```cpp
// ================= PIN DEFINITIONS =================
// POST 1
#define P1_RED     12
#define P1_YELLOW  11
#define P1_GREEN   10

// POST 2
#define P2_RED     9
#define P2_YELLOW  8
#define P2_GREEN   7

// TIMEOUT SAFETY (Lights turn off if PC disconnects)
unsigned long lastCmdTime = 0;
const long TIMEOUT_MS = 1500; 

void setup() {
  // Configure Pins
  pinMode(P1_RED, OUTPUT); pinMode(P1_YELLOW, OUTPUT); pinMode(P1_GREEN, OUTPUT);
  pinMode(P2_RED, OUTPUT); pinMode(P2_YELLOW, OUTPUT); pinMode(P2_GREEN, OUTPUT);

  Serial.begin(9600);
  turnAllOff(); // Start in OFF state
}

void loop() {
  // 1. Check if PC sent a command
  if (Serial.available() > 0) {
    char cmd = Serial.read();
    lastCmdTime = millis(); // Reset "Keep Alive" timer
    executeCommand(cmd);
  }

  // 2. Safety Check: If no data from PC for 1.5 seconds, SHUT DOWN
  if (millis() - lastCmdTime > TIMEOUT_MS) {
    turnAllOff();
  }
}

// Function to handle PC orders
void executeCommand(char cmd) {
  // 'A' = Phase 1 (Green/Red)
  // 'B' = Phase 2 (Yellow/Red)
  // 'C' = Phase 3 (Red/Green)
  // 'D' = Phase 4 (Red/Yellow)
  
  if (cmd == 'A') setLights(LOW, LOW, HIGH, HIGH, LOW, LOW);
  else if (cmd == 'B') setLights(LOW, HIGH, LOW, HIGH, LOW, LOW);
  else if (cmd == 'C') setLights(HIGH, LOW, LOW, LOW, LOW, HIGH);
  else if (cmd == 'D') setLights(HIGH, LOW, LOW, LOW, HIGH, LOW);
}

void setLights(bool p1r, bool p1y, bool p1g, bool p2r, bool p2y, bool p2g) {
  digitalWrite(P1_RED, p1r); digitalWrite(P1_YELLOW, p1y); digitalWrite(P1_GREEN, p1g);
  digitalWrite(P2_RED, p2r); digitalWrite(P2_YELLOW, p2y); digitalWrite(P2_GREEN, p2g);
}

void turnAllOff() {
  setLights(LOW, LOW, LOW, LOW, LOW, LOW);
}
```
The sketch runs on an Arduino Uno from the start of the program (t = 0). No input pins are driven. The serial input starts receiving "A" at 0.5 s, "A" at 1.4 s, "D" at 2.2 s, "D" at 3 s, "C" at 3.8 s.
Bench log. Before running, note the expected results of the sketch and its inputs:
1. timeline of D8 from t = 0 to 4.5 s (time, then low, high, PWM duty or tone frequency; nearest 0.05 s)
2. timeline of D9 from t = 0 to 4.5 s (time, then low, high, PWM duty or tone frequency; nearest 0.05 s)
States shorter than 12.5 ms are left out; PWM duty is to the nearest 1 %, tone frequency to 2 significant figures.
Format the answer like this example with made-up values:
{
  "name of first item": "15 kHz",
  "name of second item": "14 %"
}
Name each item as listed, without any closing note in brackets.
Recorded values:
{
  "timeline of D8 from t = 0 to 4.5 s": "0 s low; 2.2 s high; 3.8 s low",
  "timeline of D9 from t = 0 to 4.5 s": "0 s low; 0.5 s high; 2.2 s low"
}
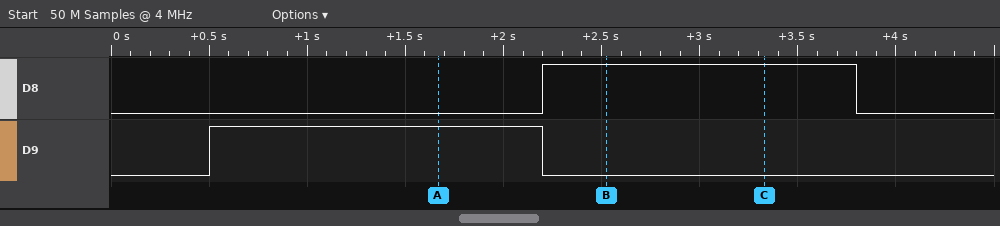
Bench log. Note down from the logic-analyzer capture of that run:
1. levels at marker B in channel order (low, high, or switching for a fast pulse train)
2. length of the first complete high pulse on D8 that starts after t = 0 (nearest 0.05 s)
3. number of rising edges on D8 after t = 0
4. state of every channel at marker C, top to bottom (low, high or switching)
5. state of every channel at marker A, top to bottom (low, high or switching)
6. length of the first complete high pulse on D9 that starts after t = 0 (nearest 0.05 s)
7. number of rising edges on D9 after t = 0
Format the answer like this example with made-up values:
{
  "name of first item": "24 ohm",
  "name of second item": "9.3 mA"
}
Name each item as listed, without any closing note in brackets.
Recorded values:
{
  "levels at marker B in channel order": "D8 high, D9 low",
  "length of the first complete high pulse on D8 that starts after t = 0": "1.60 s",
  "number of rising edges on D8 after t = 0": "1",
  "state of every channel at marker C, top to bottom": "D8 high, D9 low",
  "state of every channel at marker A, top to bottom": "D8 low, D9 high",
  "length of the first complete high pulse on D9 that starts after t = 0": "1.70 s",
  "number of rising edges on D9 after t = 0": "1"
}
